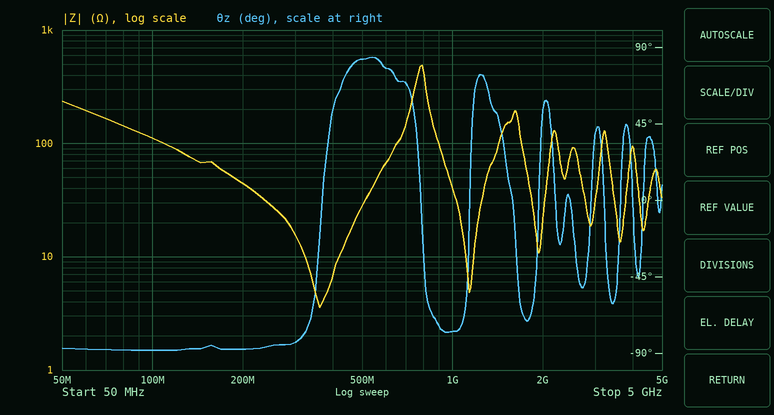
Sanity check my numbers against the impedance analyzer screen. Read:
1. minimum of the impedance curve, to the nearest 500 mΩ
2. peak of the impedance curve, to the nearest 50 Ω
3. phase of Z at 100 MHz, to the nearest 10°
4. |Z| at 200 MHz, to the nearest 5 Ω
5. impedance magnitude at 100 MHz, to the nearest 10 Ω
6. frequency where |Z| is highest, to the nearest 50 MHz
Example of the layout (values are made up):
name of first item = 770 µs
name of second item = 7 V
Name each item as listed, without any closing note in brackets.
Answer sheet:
minimum of the impedance curve, to the nearest 500 mΩ = 3.5 Ω
peak of the impedance curve, to the nearest 50 Ω = 500 Ω
phase of Z at 100 MHz, to the nearest 10° = -90°
|Z| at 200 MHz, to the nearest 5 Ω = 45 Ω
impedance magnitude at 100 MHz, to the nearest 10 Ω = 110 Ω
frequency where |Z| is highest, to the nearest 50 MHz = 800 MHz
